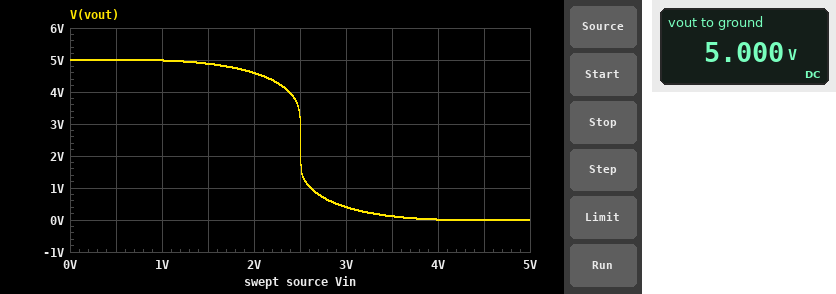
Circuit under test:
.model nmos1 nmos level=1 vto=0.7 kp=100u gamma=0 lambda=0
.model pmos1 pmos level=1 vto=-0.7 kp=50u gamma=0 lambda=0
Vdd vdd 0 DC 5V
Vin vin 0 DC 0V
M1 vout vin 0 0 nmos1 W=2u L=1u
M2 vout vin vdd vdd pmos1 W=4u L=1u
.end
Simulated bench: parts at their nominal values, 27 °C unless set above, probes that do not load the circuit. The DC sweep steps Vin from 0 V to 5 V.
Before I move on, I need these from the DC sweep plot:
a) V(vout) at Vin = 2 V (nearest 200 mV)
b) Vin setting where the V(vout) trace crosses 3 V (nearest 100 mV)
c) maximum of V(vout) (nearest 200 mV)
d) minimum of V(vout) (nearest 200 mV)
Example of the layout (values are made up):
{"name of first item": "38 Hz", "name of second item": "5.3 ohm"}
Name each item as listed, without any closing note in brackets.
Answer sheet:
{"V(vout) at Vin = 2 V": "4.6 V", "Vin setting where the V(vout) trace crosses 3 V": "2.5 V", "maximum of V(vout)": "5.0 V", "minimum of V(vout)": "0 V"}
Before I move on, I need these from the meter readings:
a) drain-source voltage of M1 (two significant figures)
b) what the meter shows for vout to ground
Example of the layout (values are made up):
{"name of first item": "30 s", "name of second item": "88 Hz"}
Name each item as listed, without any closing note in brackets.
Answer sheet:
{"drain-source voltage of M1": "5.0 V", "what the meter shows for vout to ground": "5.000 V"}
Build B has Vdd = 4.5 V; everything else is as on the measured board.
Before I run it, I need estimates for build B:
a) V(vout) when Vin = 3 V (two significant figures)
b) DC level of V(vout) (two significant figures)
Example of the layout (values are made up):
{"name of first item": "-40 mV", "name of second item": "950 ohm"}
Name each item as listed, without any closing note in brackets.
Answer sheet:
{"V(vout) when Vin = 3 V": "140 mV", "DC level of V(vout)": "4.5 V"}
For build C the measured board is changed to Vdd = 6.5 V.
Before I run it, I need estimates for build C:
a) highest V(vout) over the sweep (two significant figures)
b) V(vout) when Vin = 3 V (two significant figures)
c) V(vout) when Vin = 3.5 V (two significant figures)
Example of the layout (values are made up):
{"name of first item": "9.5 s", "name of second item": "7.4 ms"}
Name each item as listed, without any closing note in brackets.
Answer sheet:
{"highest V(vout) over the sweep": "6.5 V", "V(vout) when Vin = 3 V": "5.3 V", "V(vout) when Vin = 3.5 V": "1.2 V"}
